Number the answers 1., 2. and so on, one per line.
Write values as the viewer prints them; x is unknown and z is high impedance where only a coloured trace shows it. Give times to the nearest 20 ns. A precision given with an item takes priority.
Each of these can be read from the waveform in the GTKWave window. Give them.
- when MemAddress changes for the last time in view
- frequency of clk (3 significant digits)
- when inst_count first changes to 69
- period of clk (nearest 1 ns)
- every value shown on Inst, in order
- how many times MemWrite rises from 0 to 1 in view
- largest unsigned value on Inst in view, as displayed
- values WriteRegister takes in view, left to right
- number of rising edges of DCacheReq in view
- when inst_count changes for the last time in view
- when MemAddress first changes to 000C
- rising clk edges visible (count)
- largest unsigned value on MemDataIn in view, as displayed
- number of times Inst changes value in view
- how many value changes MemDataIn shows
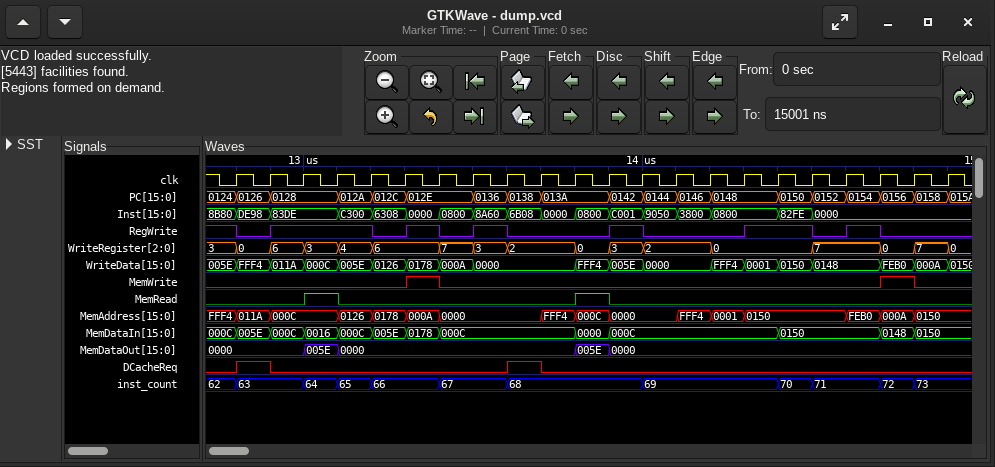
1. 14800 ns
2. 10.0 MHz
3. 14000 ns
4. 100 ns
5. 8B80, DE98, 83DE, C300, 6308, 0000, 0800, 8A60, 6B08, 0000, 0800, C001, 9050, 3800, 0800, 82FE, 0000
6. 2
7. DE98
8. 3, 0, 6, 3, 4, 6, 7, 3, 2, 0, 3, 2, 0, 7, 0, 7, 0
9. 2
10. 14800 ns
11. 12900 ns
12. 22
13. 0178
14. 16
15. 12
